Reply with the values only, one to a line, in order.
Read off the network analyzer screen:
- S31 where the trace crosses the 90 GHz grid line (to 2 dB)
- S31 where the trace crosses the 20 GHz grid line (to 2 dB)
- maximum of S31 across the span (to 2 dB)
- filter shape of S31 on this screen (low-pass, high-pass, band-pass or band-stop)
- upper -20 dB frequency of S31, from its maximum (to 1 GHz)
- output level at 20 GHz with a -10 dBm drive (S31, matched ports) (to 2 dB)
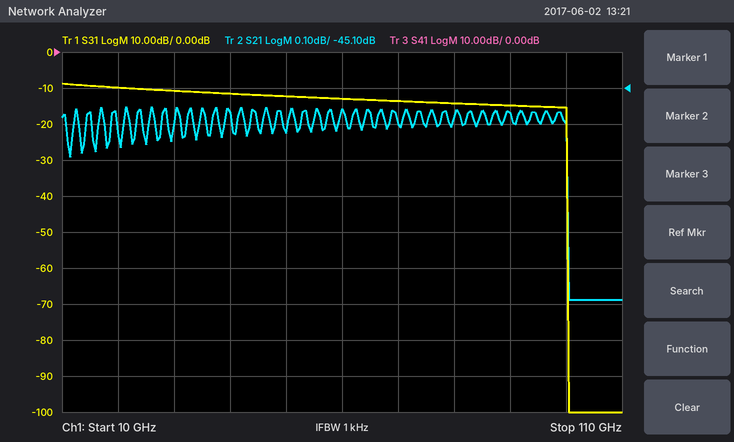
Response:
-14 dB
-10 dB
-8 dB
low-pass
100 GHz
-20 dBm
